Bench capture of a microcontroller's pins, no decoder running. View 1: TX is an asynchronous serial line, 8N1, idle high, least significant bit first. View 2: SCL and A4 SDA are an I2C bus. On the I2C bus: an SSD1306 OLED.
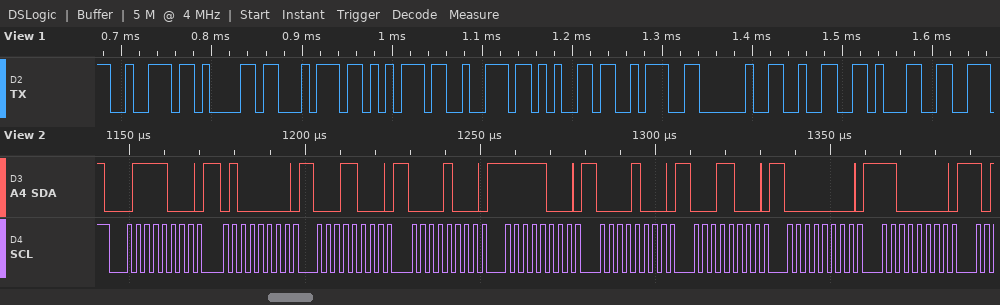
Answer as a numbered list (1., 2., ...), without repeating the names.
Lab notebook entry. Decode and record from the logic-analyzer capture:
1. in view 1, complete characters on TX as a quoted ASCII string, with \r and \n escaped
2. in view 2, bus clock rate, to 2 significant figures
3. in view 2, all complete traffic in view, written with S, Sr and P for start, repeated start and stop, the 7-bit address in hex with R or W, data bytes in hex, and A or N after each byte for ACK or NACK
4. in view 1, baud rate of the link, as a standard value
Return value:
1. "rature: 21"
2. 400 kHz
3. S 3CW A 40 A 18 A 08 A F8 A 08 A 18 A 00 A C0 A
4. 115200 baud
